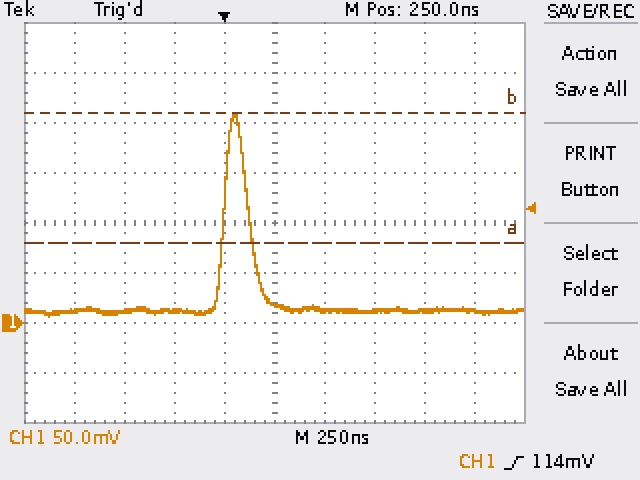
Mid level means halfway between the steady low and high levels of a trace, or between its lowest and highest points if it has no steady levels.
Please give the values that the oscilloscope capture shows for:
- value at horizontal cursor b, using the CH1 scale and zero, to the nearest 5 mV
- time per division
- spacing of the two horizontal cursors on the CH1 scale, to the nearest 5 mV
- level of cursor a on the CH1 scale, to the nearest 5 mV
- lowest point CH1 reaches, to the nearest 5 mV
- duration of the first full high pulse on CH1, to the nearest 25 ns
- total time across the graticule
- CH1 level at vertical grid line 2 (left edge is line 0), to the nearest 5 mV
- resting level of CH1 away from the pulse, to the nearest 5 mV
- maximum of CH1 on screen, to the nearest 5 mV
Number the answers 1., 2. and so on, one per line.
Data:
1. 210 mV
2. 250 ns
3. 130 mV
4. 80 mV
5. 5 mV
6. 125 ns
7. 2.5 µs
8. 10 mV
9. 10 mV
10. 210 mV
